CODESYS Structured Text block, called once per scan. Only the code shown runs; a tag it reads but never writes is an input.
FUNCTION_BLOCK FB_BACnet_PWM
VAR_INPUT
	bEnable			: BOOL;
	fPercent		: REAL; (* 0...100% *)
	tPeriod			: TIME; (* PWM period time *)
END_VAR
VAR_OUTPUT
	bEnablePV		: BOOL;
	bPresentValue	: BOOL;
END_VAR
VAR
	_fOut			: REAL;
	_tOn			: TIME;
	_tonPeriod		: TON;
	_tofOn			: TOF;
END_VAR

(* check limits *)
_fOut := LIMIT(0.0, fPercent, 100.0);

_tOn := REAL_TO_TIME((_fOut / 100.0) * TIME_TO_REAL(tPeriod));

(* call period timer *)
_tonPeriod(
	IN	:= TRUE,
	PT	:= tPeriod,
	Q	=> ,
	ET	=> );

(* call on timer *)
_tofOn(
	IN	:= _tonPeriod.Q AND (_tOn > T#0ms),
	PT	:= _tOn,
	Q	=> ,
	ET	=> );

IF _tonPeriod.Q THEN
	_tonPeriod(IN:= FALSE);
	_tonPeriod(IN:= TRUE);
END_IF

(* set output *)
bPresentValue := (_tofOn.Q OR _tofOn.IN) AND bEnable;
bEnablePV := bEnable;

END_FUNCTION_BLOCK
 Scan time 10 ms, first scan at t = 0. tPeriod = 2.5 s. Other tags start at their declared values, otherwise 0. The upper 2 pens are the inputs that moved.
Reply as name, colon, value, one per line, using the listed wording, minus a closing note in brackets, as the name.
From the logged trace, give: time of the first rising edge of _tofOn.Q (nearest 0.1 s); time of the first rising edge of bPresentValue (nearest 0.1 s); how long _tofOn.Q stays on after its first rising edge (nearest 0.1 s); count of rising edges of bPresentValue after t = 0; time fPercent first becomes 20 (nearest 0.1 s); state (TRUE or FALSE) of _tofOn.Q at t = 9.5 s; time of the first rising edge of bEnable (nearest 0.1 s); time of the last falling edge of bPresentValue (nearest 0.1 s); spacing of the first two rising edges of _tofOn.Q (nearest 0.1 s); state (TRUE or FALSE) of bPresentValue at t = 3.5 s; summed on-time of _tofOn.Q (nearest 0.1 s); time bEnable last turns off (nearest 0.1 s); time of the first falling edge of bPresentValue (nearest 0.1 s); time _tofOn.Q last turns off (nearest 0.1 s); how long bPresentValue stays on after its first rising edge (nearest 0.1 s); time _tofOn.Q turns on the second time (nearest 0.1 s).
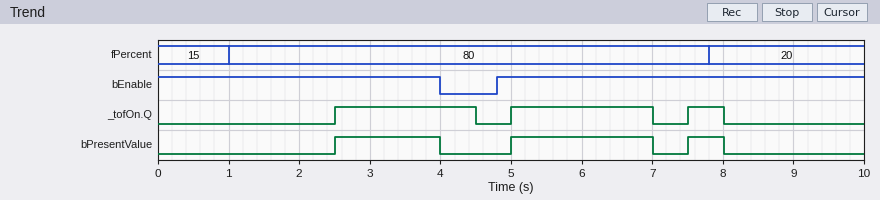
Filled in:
time of the first rising edge of _tofOn.Q: 2.5 s
time of the first rising edge of bPresentValue: 2.5 s
how long _tofOn.Q stays on after its first rising edge: 2.0 s
count of rising edges of bPresentValue after t = 0: 3
time fPercent first becomes 20: 7.8 s
state (TRUE or FALSE) of _tofOn.Q at t = 9.5 s: FALSE
time of the first rising edge of bEnable: 4.8 s
time of the last falling edge of bPresentValue: 8.0 s
spacing of the first two rising edges of _tofOn.Q: 2.5 s
state (TRUE or FALSE) of bPresentValue at t = 3.5 s: TRUE
summed on-time of _tofOn.Q: 4.5 s
time bEnable last turns off: 4.0 s
time of the first falling edge of bPresentValue: 4.0 s
time _tofOn.Q last turns off: 8.0 s
how long bPresentValue stays on after its first rising edge: 1.5 s
time _tofOn.Q turns on the second time: 5.0 s
